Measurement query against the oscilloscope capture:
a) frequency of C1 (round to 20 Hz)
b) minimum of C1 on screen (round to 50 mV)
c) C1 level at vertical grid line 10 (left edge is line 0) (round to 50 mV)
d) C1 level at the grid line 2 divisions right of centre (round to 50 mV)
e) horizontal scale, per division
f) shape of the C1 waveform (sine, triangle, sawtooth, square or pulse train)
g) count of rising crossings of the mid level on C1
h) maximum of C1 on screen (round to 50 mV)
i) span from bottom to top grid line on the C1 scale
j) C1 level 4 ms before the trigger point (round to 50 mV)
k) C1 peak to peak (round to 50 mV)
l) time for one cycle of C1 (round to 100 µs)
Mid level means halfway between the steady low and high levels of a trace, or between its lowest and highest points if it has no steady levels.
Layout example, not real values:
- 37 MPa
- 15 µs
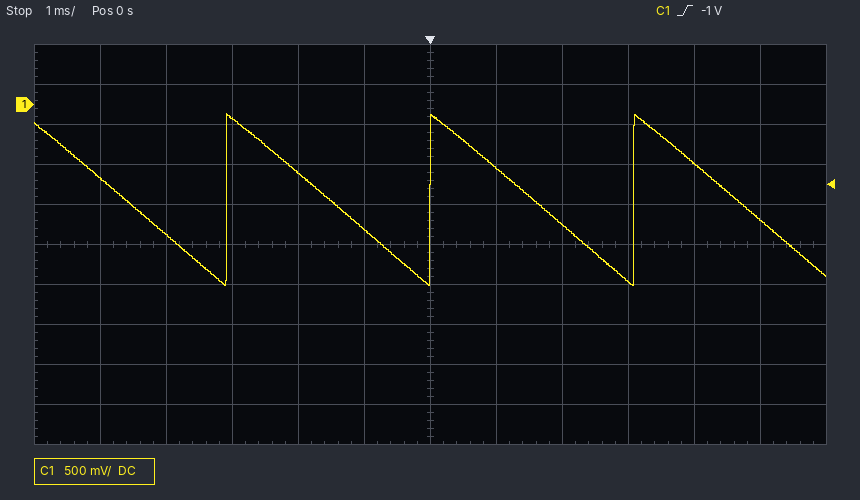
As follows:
- 320 Hz
- -2.25 V
- -750 mV
- -1.50 V
- 1 ms
- sawtooth
- 3
- -100 mV
- 5 V
- -1.65 V
- 2.15 V
- 3.1 ms
